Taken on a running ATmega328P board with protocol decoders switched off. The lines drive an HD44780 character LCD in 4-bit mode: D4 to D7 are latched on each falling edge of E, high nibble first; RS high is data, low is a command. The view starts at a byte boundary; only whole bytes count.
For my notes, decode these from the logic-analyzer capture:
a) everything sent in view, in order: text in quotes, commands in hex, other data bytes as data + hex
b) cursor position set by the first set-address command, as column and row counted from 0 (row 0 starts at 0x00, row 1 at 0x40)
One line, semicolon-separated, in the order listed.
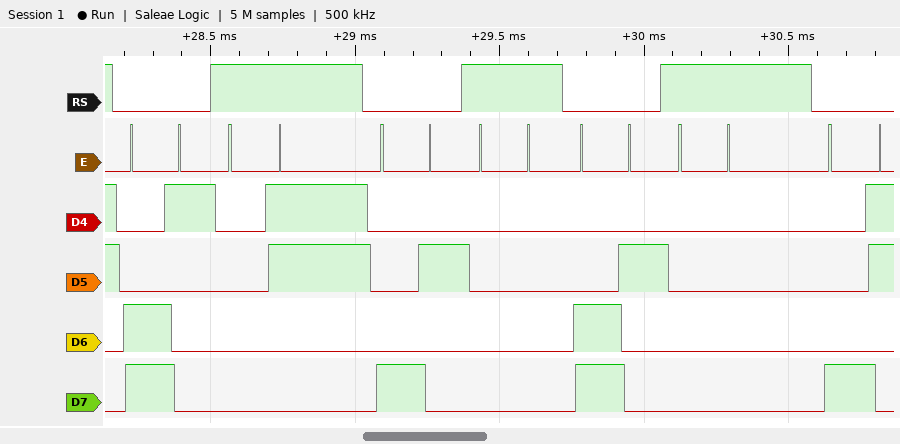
0xC1 data 03 0x82 data 00 0xC2 data 00 0x83; column 1, row 1
